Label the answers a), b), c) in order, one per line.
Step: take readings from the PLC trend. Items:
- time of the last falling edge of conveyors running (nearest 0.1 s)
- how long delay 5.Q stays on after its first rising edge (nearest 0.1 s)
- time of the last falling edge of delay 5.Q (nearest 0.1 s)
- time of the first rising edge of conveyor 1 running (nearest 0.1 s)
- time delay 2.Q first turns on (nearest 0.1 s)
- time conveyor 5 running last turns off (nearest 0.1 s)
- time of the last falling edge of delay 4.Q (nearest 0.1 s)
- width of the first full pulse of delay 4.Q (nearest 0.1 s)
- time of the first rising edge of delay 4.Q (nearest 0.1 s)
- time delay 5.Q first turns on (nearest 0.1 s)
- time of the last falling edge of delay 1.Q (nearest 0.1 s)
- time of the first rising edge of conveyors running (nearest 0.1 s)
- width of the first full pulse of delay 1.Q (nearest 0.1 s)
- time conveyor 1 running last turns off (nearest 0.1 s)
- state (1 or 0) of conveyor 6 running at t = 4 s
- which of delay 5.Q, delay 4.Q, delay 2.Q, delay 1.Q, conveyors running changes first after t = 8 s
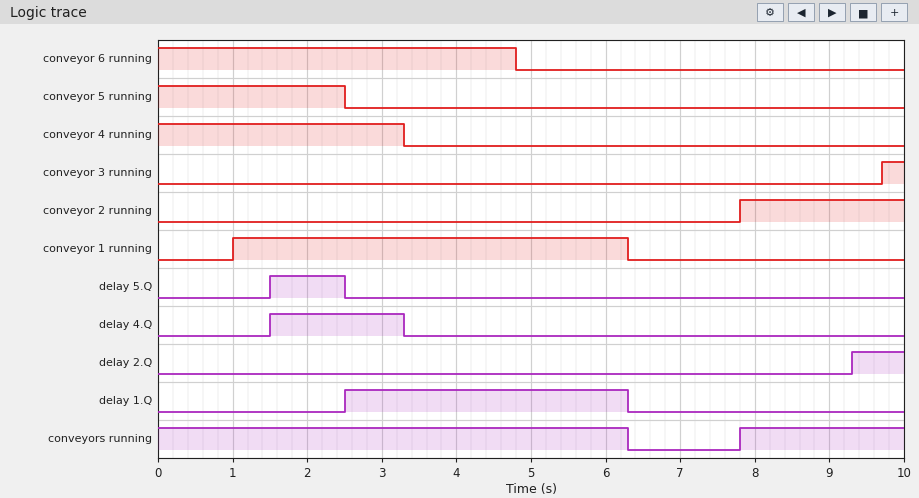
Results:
a) 6.3 s
b) 1.0 s
c) 2.5 s
d) 1.0 s
e) 9.3 s
f) 2.5 s
g) 3.3 s
h) 1.8 s
i) 1.5 s
j) 1.5 s
k) 6.3 s
l) 7.8 s
m) 3.8 s
n) 6.3 s
o) 1
p) delay 2.Q
